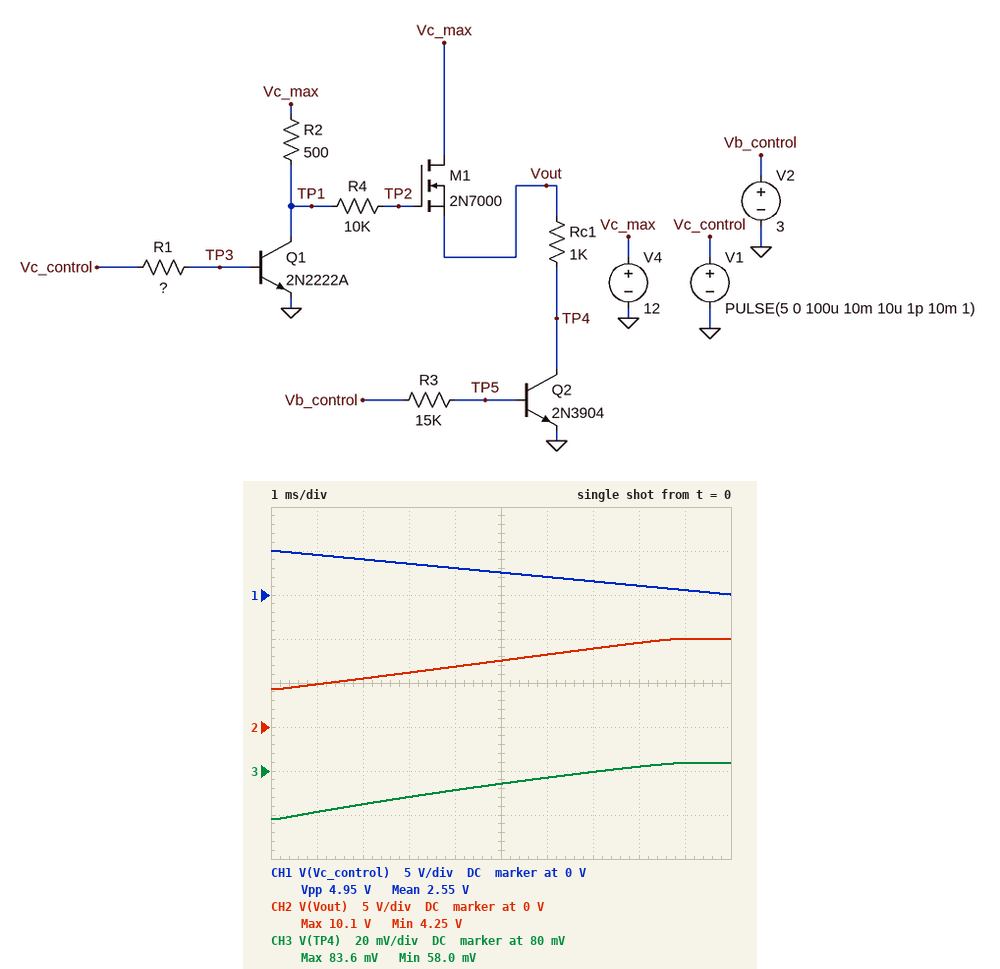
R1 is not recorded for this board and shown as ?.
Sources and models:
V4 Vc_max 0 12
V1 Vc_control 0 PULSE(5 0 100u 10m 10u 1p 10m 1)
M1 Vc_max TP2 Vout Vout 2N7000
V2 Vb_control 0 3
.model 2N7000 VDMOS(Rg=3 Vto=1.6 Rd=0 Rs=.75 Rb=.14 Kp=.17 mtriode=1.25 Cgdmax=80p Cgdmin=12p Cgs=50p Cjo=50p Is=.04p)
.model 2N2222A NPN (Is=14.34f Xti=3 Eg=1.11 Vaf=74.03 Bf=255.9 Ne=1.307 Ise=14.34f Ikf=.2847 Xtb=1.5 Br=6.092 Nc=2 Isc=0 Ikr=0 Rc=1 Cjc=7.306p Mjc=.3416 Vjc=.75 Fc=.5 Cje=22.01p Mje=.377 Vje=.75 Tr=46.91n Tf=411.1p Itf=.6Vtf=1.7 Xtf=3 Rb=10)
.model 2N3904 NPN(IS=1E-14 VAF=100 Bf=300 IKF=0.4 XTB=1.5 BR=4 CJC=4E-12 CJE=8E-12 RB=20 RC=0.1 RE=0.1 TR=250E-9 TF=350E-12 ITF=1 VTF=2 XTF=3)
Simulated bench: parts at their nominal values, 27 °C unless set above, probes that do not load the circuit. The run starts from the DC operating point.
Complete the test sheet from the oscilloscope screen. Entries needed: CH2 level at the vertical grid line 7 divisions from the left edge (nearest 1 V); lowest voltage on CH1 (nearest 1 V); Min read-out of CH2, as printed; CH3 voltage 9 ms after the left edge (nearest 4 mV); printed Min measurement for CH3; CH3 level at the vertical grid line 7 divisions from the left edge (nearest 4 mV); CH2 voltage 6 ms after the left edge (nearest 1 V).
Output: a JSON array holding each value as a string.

["9 V", "0 V", "4.25 V", "84 mV", "58.0 mV", "80 mV", "8 V"]
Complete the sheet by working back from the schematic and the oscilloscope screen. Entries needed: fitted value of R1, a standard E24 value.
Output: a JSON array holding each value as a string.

["68 kΩ"]
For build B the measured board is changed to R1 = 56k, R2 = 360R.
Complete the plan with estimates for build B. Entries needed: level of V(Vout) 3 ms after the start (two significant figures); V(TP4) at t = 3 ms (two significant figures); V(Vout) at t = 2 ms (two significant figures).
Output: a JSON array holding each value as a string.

["6.6 V", "70 mV", "6.0 V"]
